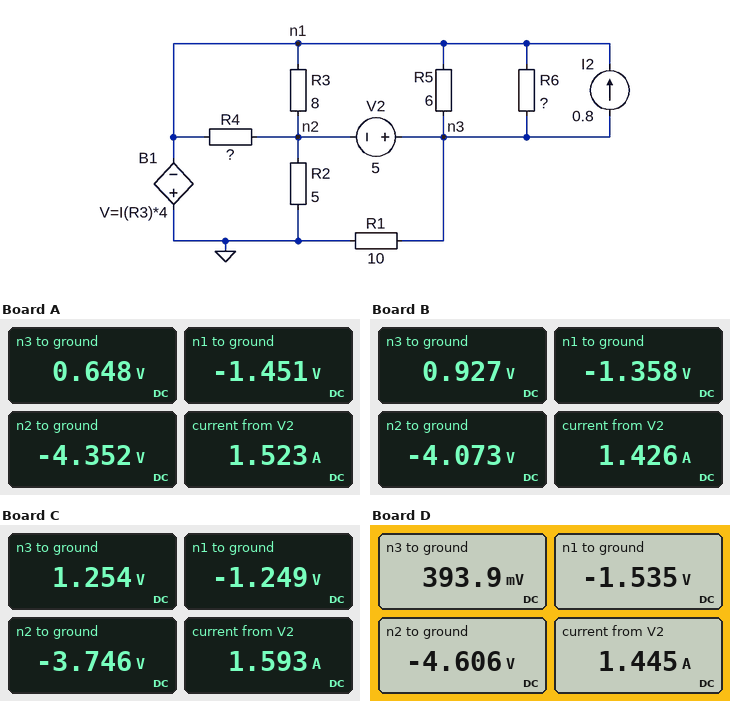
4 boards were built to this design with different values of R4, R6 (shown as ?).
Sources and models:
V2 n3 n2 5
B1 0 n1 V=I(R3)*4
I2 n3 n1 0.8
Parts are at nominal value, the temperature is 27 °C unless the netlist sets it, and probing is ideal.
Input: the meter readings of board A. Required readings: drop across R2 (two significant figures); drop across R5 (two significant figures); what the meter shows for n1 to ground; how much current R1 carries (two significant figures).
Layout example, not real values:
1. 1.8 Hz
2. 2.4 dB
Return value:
1. 4.4 V
2. 2.1 V
3. -1.451 V
4. 65 mA
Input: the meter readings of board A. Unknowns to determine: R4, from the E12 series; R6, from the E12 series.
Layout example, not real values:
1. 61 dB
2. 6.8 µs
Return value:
1. 10 Ω
2. 6.8 Ω
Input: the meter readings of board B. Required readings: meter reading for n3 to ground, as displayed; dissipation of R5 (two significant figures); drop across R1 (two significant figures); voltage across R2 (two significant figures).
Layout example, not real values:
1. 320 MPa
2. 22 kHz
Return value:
1. 0.927 V
2. 870 mW
3. 930 mV
4. 4.1 V
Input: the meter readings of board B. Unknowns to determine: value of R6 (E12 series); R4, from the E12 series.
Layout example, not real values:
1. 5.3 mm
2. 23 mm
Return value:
1. 15 Ω
2. 10 Ω
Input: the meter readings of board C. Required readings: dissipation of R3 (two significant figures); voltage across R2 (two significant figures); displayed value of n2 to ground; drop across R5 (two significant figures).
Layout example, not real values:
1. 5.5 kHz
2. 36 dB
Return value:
1. 780 mW
2. 3.7 V
3. -3.746 V
4. 2.5 V
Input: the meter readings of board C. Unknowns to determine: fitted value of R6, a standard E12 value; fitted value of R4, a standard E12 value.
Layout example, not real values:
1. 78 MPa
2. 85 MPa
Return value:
1. 10 Ω
2. 4.7 Ω
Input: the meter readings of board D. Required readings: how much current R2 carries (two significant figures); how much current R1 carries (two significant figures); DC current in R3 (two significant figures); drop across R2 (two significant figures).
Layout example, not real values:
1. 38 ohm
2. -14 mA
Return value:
1. 920 mA
2. 39 mA
3. 380 mA
4. 4.6 V
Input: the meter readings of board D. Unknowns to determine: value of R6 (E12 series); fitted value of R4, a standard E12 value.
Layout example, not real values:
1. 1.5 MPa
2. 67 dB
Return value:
1. 6.8 Ω
2. 22 Ω
